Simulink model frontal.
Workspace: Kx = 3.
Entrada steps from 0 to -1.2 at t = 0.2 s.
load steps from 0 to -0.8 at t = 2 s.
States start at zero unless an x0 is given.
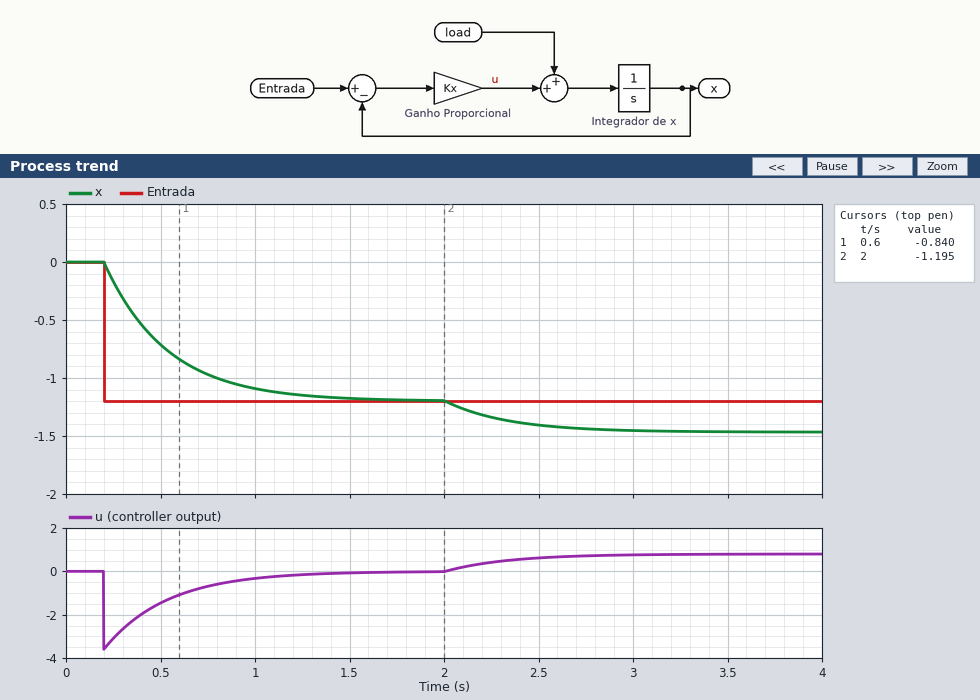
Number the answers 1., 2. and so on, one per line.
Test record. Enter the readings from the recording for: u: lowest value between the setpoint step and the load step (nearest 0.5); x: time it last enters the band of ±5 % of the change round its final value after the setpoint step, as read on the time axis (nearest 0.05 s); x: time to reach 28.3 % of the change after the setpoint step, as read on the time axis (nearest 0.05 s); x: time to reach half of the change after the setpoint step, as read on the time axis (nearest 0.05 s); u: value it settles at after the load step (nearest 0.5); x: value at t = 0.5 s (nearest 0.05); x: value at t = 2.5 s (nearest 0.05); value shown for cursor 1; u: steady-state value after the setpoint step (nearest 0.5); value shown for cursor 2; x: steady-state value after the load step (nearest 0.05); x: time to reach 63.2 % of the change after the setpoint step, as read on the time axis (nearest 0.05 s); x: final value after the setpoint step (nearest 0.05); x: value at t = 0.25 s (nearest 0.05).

1. -3.5
2. 1.20 s
3. 0.30 s
4. 0.45 s
5. 1.0
6. -0.70
7. -1.40
8. -0.840
9. 0.0
10. -1.195
11. -1.45
12. 0.55 s
13. -1.20
14. -0.15
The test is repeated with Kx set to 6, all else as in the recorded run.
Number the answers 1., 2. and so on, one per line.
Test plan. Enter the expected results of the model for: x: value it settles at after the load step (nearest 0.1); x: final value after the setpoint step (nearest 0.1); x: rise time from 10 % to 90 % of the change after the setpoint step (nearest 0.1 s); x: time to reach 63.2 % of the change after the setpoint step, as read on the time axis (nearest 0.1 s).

1. -1.3
2. -1.2
3. 0.4 s
4. 0.4 s
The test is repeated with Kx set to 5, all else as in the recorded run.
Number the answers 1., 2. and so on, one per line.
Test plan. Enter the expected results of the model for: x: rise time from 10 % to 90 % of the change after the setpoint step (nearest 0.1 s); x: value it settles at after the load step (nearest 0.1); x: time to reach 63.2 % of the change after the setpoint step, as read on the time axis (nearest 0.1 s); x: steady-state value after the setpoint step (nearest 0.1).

1. 0.4 s
2. -1.4
3. 0.4 s
4. -1.2
